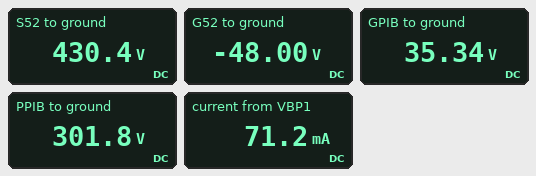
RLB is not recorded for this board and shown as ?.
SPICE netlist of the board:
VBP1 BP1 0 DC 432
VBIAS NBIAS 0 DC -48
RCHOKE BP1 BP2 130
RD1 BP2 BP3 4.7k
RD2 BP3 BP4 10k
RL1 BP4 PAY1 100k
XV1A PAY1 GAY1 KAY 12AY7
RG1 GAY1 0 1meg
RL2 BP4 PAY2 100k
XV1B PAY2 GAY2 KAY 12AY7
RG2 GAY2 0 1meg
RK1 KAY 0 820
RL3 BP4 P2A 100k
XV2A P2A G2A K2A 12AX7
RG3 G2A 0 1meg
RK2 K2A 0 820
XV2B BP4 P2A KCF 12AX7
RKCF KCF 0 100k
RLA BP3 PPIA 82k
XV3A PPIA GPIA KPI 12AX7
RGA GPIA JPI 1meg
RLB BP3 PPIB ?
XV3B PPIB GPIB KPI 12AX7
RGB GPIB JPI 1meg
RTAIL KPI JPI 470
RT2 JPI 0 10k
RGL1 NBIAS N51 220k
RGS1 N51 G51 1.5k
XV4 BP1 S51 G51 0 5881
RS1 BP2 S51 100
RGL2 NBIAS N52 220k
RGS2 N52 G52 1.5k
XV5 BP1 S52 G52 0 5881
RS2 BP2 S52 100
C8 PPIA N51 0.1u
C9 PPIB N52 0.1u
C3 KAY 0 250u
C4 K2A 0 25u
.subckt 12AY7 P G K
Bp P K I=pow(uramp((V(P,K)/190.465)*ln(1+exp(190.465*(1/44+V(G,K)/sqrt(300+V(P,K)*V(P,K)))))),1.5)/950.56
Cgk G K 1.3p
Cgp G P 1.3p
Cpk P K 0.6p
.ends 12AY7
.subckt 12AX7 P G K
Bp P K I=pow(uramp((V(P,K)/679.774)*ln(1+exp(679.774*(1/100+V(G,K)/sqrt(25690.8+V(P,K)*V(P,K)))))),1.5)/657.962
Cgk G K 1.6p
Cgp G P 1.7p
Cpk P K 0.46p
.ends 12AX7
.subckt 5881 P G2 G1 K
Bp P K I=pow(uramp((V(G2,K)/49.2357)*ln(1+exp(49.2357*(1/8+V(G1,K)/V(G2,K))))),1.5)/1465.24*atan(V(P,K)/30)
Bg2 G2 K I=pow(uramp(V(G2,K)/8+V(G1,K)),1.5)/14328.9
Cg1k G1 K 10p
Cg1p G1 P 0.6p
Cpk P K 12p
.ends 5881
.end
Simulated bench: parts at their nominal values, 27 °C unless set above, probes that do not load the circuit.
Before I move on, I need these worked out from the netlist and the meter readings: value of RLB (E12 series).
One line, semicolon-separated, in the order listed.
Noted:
39 kΩ
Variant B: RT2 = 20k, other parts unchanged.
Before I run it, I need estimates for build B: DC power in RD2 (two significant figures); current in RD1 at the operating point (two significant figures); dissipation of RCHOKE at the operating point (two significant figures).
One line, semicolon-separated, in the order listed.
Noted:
410 mW; 9.6 mA; 17 mW
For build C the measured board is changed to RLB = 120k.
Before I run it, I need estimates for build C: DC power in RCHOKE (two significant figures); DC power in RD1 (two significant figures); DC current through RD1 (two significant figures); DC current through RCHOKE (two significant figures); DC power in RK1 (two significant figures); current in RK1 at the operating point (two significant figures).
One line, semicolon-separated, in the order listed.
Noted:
17 mW; 410 mW; 9.4 mA; 11 mA; 8.2 mW; 3.2 mA
